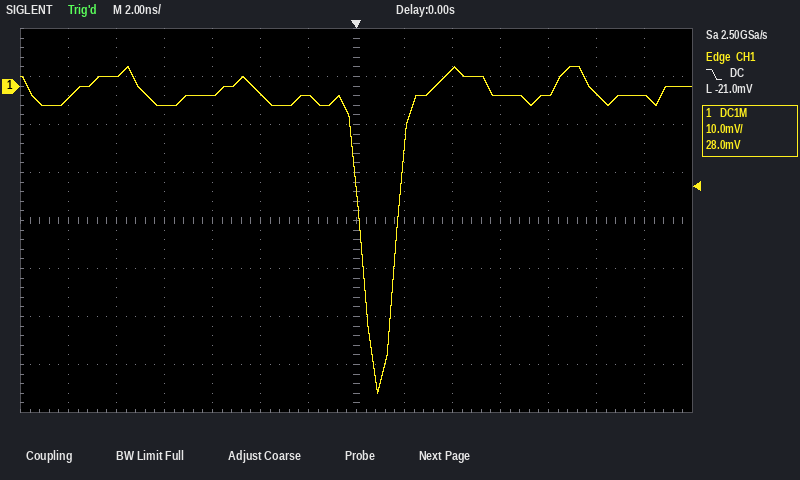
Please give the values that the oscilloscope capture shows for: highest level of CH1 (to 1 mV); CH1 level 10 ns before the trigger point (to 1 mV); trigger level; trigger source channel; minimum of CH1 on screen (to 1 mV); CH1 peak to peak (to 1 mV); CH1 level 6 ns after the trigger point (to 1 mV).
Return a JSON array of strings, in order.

["4 mV", "2 mV", "-21.0 mV", "CH1", "-64 mV", "68 mV", "-2 mV"]
